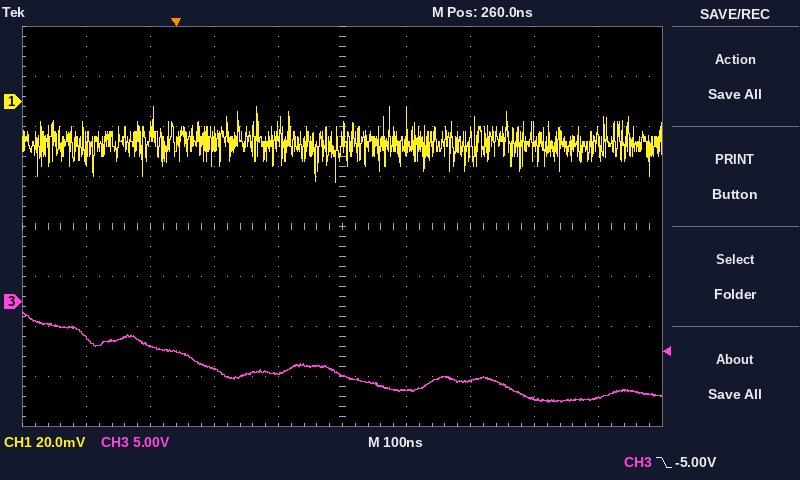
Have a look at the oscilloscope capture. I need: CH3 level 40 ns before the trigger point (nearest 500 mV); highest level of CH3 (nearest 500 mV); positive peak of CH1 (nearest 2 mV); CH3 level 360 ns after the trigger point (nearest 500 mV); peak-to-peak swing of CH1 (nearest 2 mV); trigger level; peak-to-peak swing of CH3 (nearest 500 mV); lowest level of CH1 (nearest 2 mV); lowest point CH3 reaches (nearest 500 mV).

-4.5 V
-1.0 V
-2 mV
-9.0 V
30 mV
-5.00 V
9.0 V
-32 mV
-10.0 V
